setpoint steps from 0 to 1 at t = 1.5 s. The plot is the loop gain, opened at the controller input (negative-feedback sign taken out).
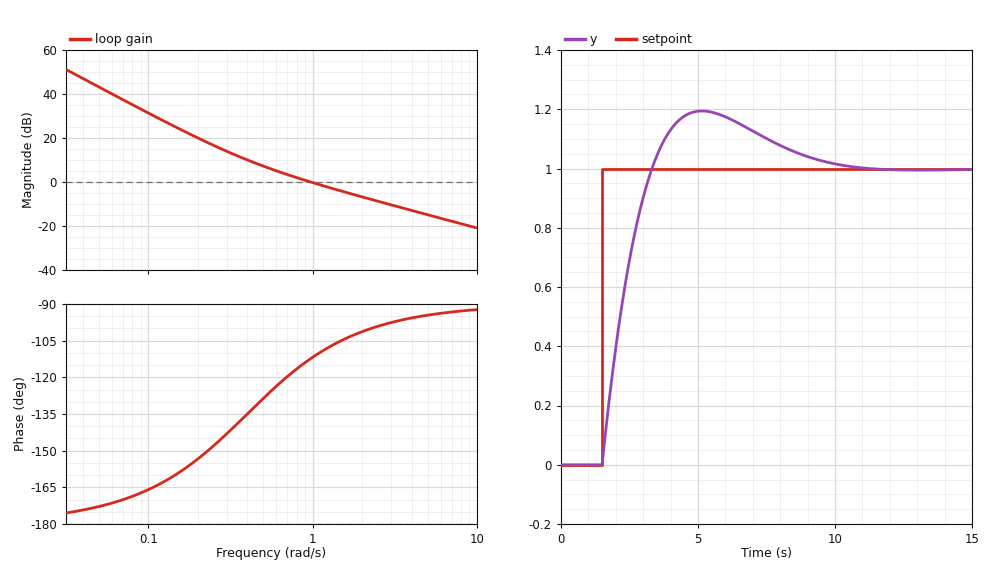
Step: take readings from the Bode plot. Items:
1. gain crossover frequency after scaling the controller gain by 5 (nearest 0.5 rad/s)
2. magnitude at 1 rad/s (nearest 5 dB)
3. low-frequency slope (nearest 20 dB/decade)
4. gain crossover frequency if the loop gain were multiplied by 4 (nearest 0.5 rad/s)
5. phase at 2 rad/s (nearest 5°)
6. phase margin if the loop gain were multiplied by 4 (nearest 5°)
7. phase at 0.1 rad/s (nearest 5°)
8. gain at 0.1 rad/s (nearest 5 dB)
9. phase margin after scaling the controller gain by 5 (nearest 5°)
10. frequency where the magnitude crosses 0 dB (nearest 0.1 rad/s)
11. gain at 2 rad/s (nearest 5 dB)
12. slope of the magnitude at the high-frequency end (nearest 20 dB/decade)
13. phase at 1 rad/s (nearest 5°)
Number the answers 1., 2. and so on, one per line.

1. 4.5 rad/s
2. 0 dB
3. -40 dB/decade
4. 3.5 rad/s
5. -100°
6. 85°
7. -165°
8. 30 dB
9. 85°
10. 1.0 rad/s
11. -5 dB
12. -20 dB/decade
13. -110°
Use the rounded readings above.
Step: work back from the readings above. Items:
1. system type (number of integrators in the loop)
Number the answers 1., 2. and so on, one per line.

1. 2
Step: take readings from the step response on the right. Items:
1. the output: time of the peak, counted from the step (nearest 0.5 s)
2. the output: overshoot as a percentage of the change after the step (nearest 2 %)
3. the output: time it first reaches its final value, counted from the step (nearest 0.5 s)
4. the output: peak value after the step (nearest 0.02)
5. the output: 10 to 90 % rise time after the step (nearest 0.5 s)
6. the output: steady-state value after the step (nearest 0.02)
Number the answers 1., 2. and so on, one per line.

1. 3.5 s
2. 20 %
3. 2.0 s
4. 1.20
5. 1.5 s
6. 1.00
